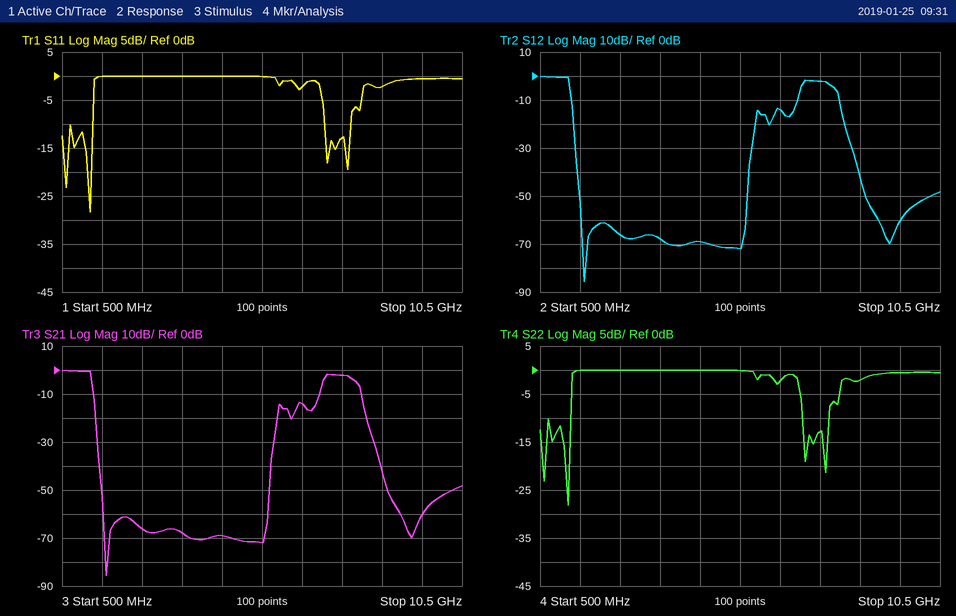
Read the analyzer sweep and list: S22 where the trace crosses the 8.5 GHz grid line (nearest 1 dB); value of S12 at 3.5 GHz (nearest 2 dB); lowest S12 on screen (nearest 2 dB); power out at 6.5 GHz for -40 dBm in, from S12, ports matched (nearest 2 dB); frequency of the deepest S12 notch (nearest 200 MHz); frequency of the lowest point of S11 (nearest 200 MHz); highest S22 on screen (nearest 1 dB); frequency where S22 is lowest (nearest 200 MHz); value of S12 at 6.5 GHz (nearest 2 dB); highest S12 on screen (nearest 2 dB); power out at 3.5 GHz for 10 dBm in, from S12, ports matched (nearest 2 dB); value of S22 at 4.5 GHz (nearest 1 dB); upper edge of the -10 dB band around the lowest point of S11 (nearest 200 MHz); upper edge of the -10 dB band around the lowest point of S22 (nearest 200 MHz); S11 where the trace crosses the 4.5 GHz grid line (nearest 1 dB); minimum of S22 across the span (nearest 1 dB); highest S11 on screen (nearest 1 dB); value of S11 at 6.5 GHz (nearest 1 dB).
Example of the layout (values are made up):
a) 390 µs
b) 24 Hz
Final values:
a) -2 dB
b) -68 dB
c) -86 dB
d) -54 dBm
e) 1.6 GHz
f) 1.2 GHz
g) 0 dB
h) 1.2 GHz
i) -14 dB
j) 0 dB
k) -58 dBm
l) 0 dB
m) 1.2 GHz
n) 1.2 GHz
o) 0 dB
p) -28 dB
q) 0 dB
r) -2 dB
